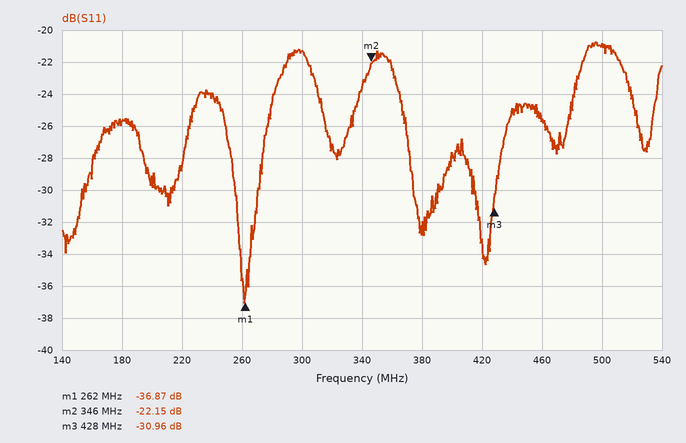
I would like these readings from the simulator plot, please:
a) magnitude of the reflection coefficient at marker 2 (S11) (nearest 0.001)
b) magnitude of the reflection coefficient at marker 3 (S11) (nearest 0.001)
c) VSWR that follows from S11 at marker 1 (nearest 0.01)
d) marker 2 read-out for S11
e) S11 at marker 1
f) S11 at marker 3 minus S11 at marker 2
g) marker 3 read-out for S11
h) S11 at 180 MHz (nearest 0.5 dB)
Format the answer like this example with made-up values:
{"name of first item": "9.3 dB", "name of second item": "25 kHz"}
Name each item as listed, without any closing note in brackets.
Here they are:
{"magnitude of the reflection coefficient at marker 2 (S11)": "0.078", "magnitude of the reflection coefficient at marker 3 (S11)": "0.028", "VSWR that follows from S11 at marker 1": "1.03", "marker 2 read-out for S11": "-22.15 dB", "S11 at marker 1": "-36.87 dB", "S11 at marker 3 minus S11 at marker 2": "-8.81 dB", "marker 3 read-out for S11": "-30.96 dB", "S11 at 180 MHz": "-25.5 dB"}
